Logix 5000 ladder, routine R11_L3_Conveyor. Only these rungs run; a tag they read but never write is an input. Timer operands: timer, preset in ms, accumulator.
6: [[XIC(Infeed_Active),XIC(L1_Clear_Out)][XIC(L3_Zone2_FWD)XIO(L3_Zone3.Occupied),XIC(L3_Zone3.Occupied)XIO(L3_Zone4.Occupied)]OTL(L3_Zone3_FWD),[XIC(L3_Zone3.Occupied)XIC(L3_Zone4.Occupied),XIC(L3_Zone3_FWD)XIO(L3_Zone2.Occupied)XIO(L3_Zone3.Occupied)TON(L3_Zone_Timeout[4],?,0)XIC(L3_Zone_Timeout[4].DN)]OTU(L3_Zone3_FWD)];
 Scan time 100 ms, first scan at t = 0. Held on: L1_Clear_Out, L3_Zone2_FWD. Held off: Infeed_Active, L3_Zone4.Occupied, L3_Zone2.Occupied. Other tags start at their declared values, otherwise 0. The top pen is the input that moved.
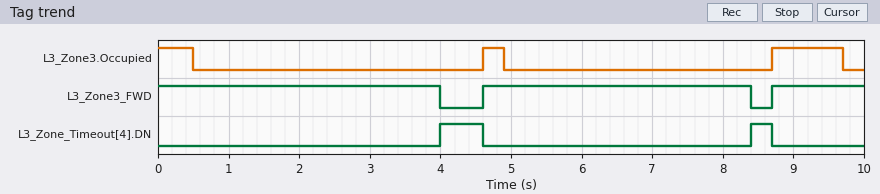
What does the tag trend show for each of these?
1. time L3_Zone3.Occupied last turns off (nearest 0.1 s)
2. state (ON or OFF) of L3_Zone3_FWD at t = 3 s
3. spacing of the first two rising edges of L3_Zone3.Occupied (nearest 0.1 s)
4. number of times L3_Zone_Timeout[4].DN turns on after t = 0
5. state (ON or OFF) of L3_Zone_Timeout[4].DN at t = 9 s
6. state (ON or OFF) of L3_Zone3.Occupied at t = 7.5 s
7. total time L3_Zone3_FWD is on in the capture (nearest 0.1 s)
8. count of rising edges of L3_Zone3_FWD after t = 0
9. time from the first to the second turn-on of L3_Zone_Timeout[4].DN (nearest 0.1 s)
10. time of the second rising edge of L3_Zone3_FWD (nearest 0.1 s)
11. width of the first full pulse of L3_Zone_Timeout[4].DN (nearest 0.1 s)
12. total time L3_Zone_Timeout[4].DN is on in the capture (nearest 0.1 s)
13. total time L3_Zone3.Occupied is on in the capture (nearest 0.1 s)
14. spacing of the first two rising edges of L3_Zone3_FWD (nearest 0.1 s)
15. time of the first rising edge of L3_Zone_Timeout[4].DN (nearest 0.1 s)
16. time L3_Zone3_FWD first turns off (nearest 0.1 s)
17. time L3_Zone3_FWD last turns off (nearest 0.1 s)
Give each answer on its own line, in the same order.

9.7 s
ON
4.1 s
2
OFF
OFF
9.1 s
2
4.4 s
8.7 s
0.6 s
0.9 s
1.8 s
4.1 s
4.0 s
4.0 s
8.4 s
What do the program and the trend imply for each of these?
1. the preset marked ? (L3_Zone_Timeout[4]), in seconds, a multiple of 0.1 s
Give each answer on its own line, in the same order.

3.5 s
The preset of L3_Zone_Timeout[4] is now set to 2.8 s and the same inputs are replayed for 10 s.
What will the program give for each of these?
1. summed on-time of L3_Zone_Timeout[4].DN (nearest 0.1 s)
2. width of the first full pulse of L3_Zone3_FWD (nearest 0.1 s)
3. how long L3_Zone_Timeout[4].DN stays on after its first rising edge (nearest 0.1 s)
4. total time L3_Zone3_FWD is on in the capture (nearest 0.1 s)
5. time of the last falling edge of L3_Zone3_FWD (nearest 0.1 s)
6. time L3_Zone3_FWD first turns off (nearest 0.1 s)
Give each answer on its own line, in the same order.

2.3 s
3.1 s
1.3 s
7.7 s
7.7 s
3.3 s
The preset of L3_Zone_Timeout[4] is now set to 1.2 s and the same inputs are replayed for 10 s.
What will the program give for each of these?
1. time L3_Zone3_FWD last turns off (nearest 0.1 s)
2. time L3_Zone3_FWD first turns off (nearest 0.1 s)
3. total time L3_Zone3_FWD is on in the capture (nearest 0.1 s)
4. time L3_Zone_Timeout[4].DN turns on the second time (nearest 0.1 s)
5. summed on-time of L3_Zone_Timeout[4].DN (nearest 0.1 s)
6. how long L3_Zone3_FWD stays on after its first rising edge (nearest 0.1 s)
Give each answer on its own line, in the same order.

6.1 s
1.7 s
4.5 s
6.1 s
5.5 s
1.5 s
